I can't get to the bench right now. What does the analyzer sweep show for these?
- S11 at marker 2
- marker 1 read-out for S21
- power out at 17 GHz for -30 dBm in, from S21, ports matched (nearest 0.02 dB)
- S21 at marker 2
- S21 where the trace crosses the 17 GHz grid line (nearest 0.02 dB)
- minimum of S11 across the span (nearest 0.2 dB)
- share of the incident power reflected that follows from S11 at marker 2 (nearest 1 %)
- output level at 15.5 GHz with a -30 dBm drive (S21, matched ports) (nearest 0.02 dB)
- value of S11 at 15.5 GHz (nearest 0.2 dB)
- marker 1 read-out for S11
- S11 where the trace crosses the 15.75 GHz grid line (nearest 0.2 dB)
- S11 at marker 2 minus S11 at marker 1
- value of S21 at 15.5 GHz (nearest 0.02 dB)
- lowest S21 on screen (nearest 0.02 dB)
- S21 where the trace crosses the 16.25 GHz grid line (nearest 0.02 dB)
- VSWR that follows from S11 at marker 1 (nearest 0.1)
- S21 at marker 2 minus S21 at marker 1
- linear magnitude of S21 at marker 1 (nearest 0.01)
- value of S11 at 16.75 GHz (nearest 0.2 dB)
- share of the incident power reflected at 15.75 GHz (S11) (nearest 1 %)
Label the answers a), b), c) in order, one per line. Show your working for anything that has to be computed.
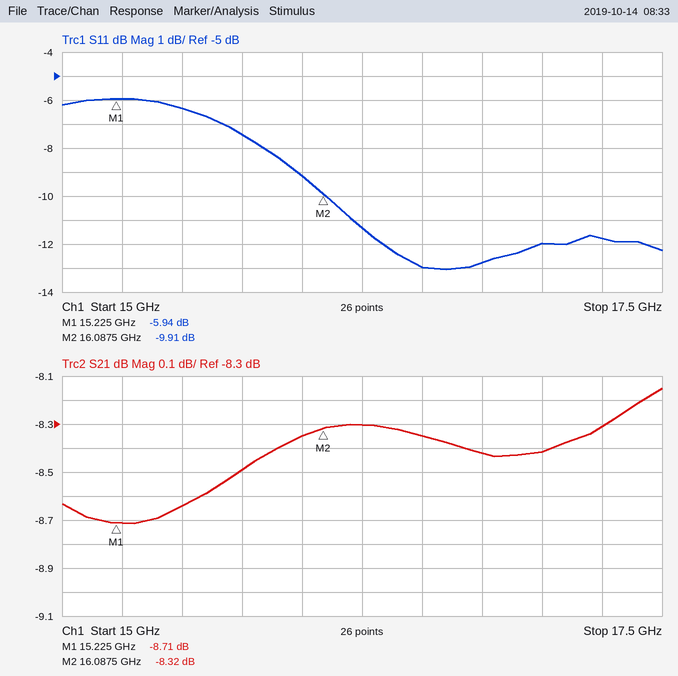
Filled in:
a) -9.91 dB
b) -8.71 dB
c) -30 dBm + (-8.42 dB) = -38.42 dBm
d) -8.32 dB
e) -8.42 dB
f) -13.0 dB
g) 10^(-9.91/10) ≈ 10 %
h) -30 dBm + (-8.64 dB) = -38.64 dBm
i) -6.4 dB
j) -5.94 dB
k) -7.4 dB
l) -9.91 − (-5.94) = -3.97 dB
m) -8.64 dB
n) -8.72 dB
o) -8.30 dB
p) (1 + 0.5047)/(1 − 0.5047) ≈ 3.0
q) -8.32 − (-8.71) = 0.39 dB
r) 10^(-8.71/20) ≈ 0.37
s) -12.8 dB
t) 10^(-7.4/10) ≈ 18 %
